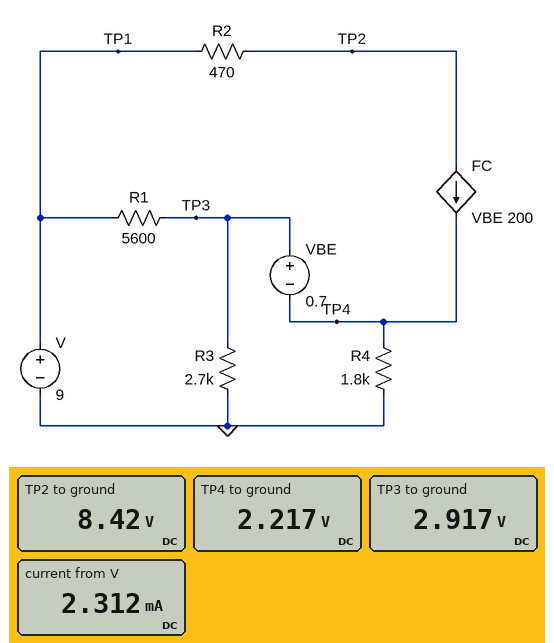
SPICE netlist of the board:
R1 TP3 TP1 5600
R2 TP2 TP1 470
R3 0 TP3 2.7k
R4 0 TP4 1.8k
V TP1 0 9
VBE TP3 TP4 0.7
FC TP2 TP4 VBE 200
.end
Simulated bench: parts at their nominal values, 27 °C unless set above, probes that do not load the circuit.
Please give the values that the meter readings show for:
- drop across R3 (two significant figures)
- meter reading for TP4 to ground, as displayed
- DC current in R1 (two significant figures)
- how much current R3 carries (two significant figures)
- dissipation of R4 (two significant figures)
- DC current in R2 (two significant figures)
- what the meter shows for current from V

2.9 V
2.217 V
1.1 mA
1.1 mA
2.7 mW
1.2 mA
2.312 mA
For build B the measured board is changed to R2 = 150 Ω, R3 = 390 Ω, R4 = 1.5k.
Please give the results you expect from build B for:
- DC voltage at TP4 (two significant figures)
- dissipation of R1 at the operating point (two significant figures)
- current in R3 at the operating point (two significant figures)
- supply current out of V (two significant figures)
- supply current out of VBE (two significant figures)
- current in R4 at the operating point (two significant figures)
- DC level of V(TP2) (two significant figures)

-110 mV
13 mW
1.5 mA
1.4 mA
380 nA
76 µA
9.0 V
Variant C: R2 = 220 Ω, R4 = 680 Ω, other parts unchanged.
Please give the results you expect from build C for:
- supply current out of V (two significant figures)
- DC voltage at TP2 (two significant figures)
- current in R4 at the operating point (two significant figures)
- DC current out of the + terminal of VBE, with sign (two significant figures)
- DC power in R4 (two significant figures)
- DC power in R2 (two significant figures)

4.3 mA
8.3 V
3.2 mA
-16 µA
7.1 mW
2.3 mW
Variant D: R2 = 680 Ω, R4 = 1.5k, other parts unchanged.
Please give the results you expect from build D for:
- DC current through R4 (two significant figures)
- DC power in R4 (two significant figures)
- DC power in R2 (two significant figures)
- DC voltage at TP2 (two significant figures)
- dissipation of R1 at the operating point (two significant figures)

1.5 mA
3.3 mW
1.5 mW
8.0 V
6.6 mW
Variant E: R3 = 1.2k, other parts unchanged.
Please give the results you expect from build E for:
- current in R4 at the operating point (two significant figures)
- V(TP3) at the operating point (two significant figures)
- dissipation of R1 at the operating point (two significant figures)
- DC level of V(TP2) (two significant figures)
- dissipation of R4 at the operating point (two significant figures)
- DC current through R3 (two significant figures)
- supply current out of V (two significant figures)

490 µA
1.6 V
9.8 mW
8.8 V
440 µW
1.3 mA
1.8 mA
